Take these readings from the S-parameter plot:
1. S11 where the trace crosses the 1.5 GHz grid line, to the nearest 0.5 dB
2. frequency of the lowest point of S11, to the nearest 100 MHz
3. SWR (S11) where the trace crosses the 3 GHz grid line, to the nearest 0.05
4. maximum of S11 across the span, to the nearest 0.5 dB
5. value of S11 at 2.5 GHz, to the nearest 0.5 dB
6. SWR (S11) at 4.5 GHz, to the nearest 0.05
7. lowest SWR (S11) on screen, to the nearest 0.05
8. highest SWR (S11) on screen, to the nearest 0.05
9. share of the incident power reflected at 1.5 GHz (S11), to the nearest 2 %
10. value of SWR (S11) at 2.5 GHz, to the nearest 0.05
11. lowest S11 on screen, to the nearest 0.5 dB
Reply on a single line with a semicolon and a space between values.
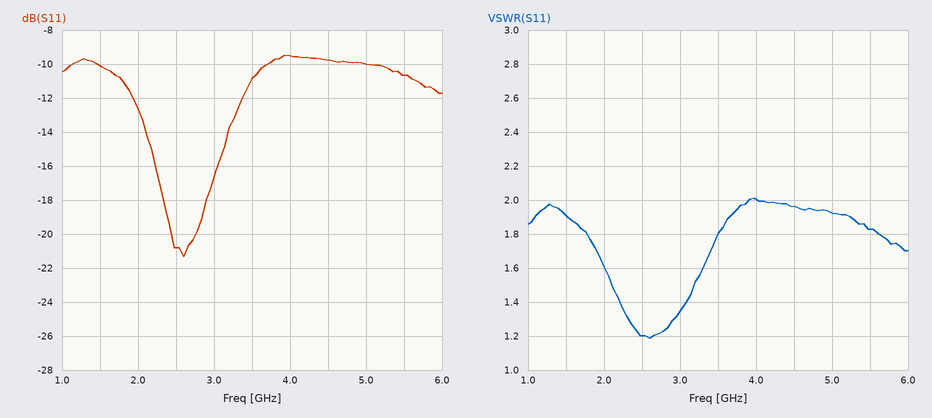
-10.0 dB; 2.6 GHz; 1.35; -9.5 dB; -21.0 dB; 1.95; 1.20; 2.00; 10 %; 1.20; -21.5 dB
